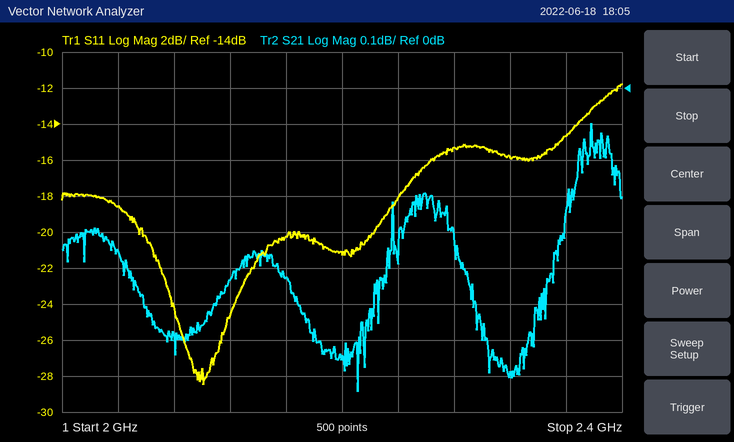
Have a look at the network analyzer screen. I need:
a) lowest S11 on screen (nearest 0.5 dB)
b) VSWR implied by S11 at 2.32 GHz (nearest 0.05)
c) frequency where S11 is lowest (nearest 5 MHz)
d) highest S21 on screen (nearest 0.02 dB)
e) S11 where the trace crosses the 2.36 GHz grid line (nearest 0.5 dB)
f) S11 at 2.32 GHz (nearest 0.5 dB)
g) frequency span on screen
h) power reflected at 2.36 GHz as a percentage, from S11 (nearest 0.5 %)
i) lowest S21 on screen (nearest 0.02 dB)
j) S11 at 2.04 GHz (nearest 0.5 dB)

-28.5 dB
1.40
2.100 GHz
-0.10 dB
-14.5 dB
-16.0 dB
400 MHz
3.5 %
-0.84 dB
-18.5 dB
